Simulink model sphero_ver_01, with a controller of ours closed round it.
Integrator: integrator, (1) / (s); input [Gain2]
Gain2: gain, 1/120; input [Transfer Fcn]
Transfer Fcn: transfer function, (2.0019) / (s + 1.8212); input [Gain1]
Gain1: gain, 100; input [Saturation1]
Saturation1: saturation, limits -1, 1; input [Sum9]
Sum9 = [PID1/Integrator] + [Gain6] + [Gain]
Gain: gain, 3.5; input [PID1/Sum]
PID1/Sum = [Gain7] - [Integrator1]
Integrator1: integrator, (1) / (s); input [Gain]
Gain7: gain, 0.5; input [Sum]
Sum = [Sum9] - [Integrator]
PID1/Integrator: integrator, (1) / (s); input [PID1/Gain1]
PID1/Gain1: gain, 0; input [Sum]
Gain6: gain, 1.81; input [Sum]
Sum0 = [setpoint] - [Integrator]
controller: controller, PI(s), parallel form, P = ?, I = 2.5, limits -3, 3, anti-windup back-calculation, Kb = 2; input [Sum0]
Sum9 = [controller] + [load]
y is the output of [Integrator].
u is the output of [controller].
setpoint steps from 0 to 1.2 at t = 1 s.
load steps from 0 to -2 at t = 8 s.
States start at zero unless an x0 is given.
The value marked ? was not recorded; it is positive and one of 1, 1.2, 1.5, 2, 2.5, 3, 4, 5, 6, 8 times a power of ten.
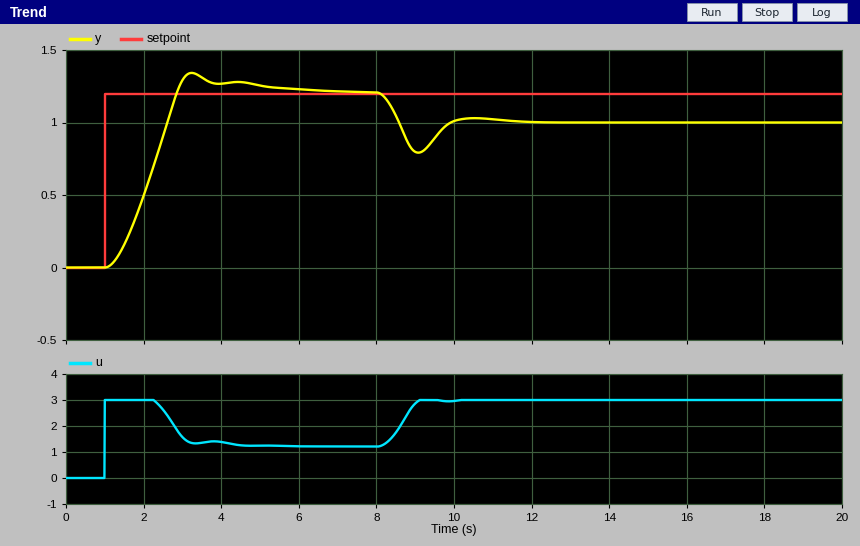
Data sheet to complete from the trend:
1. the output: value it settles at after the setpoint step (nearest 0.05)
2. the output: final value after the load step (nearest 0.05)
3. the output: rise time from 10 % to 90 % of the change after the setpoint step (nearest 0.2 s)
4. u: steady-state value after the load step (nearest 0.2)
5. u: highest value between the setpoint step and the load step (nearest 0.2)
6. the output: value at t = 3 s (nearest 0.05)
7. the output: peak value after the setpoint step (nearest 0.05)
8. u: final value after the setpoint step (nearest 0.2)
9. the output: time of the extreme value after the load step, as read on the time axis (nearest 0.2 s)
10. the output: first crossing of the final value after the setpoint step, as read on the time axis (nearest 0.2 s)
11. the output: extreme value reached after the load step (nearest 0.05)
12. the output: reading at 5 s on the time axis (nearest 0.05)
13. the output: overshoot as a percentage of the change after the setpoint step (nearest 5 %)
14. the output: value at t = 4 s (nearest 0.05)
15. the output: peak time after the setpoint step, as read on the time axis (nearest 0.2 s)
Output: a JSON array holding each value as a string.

["1.20", "1.00", "1.2 s", "3.0", "3.0", "1.30", "1.35", "1.2", "9.0 s", "2.8 s", "0.80", "1.25", "10 %", "1.25", "3.2 s"]
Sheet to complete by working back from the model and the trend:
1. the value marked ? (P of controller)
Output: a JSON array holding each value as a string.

["3"]
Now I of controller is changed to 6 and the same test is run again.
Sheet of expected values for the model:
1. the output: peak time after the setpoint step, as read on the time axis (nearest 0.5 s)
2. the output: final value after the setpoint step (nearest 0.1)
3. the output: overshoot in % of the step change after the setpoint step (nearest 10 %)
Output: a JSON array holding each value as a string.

["3.5 s", "1.2", "30 %"]
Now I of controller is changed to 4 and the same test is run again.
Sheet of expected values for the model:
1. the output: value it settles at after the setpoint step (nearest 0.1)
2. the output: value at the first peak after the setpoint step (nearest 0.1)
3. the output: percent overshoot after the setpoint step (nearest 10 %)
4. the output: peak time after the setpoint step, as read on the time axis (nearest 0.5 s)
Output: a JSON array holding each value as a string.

["1.2", "1.5", "20 %", "3.5 s"]
